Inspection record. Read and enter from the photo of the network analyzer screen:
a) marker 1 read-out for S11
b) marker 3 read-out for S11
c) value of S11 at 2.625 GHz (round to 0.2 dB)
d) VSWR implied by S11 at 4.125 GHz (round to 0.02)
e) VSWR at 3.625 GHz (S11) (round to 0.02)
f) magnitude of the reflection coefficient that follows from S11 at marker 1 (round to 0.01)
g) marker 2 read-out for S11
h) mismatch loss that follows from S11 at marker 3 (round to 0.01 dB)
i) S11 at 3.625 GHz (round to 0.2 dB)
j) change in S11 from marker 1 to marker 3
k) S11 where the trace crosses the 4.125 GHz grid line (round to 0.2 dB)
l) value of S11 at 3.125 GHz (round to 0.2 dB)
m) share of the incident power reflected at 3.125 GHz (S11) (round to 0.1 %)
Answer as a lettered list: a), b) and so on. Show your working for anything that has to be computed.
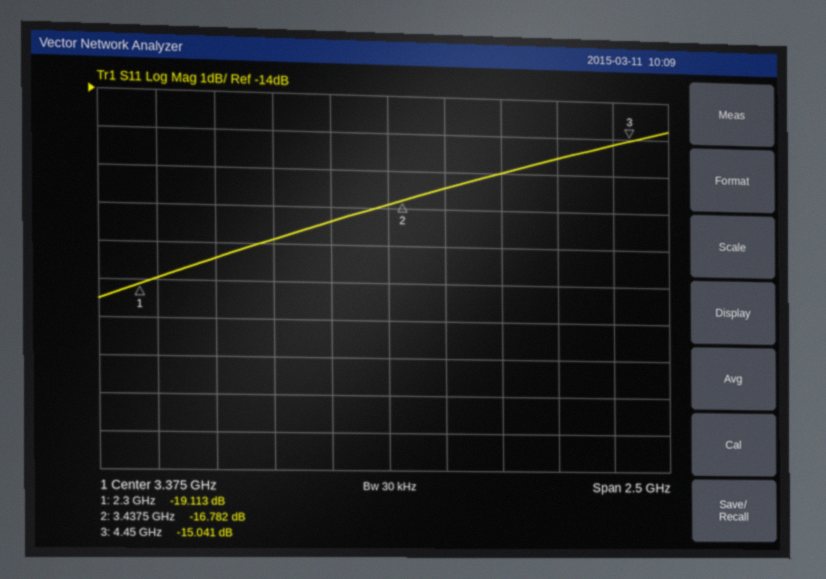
a) -19.113 dB
b) -15.041 dB
c) -18.4 dB
d) |Γ| = 10^(-15.6/20) = 0.1660; VSWR = (1 + 0.1660)/(1 − 0.1660) ≈ 1.40
e) |Γ| = 10^(-16.4/20) = 0.1514; VSWR = (1 + 0.1514)/(1 − 0.1514) ≈ 1.36
f) 10^(-19.113/20) ≈ 0.11
g) -16.782 dB
h) −10 log10(1 − 10^(-15.041/10)) ≈ 0.14 dB
i) -16.4 dB
j) -15.041 − (-19.113) = 4.072 dB
k) -15.6 dB
l) -17.4 dB
m) 10^(-17.4/10) ≈ 1.8 %
